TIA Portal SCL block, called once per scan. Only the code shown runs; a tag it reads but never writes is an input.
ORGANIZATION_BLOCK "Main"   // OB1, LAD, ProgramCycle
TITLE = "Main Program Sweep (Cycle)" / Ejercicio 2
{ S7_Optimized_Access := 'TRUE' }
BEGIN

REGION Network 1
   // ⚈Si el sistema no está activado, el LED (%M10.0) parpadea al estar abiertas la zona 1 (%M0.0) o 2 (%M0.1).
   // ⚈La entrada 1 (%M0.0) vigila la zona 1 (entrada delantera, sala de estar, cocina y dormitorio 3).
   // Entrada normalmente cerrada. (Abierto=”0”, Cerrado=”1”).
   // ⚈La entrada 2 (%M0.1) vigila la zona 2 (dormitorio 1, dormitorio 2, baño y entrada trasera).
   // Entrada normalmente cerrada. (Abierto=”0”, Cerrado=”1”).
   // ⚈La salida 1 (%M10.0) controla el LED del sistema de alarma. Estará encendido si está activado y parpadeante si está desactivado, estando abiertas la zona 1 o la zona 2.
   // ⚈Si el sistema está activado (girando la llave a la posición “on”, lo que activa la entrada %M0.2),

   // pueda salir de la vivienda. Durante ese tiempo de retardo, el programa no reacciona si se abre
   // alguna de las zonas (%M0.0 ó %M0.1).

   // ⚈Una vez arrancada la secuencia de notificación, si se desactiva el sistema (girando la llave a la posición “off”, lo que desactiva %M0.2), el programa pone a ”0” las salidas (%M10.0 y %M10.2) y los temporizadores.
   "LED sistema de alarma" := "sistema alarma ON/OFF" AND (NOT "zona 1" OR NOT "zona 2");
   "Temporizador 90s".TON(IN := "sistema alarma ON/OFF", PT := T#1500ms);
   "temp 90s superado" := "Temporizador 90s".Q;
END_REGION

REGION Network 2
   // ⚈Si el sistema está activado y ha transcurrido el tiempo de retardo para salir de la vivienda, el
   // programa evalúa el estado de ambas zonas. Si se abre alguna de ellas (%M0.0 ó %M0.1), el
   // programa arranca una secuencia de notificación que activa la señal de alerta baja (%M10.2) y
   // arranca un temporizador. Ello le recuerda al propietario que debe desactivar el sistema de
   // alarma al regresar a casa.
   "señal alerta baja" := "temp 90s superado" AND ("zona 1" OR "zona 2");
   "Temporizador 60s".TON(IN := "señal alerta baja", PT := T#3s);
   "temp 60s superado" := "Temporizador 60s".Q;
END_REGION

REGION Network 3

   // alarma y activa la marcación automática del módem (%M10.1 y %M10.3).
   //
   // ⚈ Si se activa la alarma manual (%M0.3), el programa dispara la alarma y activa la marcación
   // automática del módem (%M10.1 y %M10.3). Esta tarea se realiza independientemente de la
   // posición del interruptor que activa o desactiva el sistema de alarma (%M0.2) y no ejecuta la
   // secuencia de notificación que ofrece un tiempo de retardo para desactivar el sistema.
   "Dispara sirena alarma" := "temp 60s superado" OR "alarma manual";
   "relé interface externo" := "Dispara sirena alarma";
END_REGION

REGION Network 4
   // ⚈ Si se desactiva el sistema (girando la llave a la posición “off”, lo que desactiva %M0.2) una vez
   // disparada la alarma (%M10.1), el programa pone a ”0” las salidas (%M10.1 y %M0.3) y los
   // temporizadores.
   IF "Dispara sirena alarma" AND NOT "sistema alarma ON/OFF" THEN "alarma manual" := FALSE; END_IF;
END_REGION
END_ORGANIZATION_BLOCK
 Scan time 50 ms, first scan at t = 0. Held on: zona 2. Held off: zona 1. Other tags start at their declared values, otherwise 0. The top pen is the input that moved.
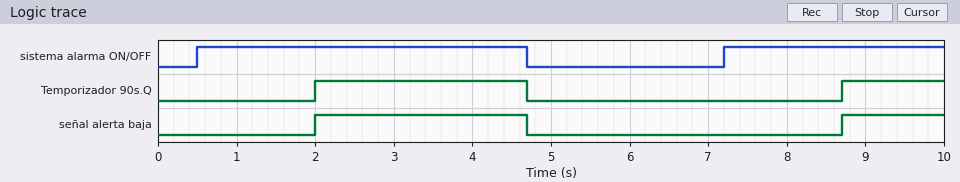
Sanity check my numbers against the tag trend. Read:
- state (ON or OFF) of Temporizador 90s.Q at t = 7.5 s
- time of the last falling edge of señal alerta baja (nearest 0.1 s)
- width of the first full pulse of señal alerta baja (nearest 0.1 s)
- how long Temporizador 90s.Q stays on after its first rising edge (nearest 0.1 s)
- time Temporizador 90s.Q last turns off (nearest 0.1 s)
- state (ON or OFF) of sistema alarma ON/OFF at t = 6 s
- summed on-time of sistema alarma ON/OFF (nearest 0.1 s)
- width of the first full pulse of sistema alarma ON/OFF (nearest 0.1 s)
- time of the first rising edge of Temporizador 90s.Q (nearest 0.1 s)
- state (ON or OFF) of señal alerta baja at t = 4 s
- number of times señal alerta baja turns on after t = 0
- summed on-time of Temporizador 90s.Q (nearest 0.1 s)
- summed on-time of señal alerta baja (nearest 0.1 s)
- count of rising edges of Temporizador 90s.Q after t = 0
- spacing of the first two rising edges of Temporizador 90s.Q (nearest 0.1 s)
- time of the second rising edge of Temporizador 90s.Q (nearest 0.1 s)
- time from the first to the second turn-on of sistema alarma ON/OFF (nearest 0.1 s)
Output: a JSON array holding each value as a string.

["OFF", "4.7 s", "2.7 s", "2.7 s", "4.7 s", "OFF", "7.0 s", "4.2 s", "2.0 s", "ON", "2", "4.0 s", "4.0 s", "2", "6.7 s", "8.7 s", "6.7 s"]
